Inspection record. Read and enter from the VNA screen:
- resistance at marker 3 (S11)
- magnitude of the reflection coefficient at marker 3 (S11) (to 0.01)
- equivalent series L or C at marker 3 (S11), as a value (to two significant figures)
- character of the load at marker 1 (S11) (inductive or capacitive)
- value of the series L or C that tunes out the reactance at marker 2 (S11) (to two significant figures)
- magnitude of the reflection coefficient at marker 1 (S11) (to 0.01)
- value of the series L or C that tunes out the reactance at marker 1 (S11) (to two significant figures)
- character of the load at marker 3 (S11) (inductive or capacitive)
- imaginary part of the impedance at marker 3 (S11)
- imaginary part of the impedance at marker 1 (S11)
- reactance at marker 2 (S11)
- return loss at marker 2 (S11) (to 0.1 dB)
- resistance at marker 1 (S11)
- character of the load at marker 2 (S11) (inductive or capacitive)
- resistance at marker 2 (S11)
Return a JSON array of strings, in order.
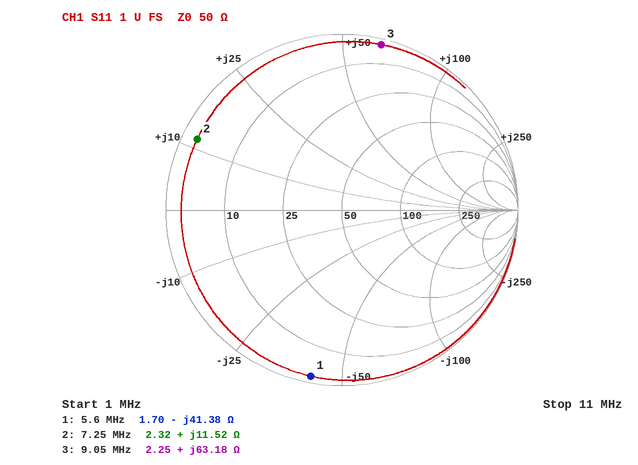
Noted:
["2.25 Ω", "0.97", "1.1 µH", "capacitive", "1.9 nF", "0.96", "1.2 µH", "inductive", "+63.18 Ω", "-41.38 Ω", "+11.52 Ω", "0.8 dB", "1.70 Ω", "inductive", "2.32 Ω"]
